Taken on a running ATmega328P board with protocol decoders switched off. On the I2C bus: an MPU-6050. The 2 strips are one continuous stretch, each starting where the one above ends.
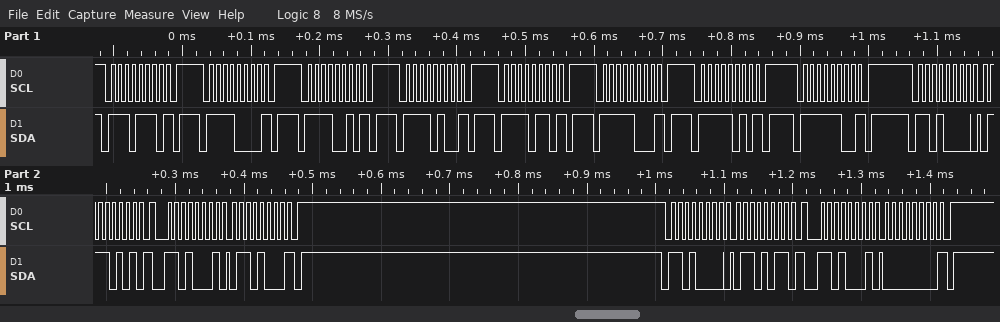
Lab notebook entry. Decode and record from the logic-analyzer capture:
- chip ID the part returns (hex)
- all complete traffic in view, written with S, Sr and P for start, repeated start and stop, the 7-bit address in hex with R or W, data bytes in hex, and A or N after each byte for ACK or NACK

0x68
S 77W N P S 78W N P S 79W N P S 7AW N P S 7BW N P S 7CW N P S 7DW N P S 7EW N P S 68W A 75 A Sr 68R A 68 N P S 68W A 6B A Sr 68R A 00 N P
